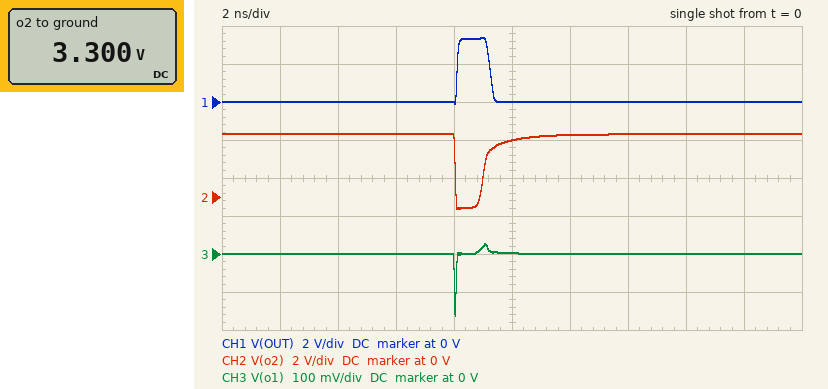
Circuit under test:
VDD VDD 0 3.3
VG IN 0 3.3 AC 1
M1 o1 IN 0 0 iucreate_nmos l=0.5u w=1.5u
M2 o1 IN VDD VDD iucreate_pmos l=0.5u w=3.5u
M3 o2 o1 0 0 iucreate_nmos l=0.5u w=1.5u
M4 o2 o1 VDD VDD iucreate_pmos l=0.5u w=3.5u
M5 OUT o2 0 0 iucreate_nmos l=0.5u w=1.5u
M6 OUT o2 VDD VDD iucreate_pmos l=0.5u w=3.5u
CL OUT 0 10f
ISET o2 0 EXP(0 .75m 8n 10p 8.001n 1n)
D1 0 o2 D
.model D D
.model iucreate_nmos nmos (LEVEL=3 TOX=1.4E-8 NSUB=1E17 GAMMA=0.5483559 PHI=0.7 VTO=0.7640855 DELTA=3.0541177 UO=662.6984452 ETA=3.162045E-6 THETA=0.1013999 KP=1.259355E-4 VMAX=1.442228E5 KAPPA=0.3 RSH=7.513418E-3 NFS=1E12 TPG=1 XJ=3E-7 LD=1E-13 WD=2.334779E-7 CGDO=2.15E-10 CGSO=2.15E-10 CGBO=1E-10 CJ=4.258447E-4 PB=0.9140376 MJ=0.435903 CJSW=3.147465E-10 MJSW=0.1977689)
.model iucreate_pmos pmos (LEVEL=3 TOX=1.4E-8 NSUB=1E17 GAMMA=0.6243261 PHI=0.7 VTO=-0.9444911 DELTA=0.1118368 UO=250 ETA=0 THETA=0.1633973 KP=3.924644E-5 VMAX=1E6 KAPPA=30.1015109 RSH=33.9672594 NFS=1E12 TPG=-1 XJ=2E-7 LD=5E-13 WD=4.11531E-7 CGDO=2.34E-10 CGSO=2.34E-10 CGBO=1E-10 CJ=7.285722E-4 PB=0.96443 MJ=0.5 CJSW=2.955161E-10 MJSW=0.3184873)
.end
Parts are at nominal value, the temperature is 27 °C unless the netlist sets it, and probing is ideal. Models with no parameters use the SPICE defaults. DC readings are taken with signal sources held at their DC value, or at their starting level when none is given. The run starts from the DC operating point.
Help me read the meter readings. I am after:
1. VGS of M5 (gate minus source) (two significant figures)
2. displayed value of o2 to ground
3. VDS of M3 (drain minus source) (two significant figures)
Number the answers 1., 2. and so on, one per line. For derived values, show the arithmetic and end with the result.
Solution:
1. 3.3 V = 3.3 V
2. 3.300 V
3. 3.3 V = 3.3 V
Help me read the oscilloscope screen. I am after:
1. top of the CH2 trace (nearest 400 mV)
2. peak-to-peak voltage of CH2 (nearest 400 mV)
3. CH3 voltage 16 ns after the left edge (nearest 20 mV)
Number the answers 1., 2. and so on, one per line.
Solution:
1. 3.2 V
2. 4.0 V
3. 0 V
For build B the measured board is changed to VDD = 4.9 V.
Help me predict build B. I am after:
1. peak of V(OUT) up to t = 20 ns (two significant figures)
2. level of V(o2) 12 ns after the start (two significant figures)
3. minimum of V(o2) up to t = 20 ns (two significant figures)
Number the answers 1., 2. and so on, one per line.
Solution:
1. 240 mV
2. 4.9 V
3. 2.9 V
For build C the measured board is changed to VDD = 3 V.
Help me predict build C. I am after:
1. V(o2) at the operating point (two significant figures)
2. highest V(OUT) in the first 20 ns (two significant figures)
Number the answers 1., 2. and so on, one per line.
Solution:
1. 3.0 V
2. 3.1 V
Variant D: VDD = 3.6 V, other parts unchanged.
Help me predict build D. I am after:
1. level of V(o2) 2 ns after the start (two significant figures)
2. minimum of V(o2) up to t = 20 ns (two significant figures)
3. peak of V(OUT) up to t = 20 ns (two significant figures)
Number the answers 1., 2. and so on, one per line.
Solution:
1. 3.6 V
2. -590 mV
3. 3.7 V
